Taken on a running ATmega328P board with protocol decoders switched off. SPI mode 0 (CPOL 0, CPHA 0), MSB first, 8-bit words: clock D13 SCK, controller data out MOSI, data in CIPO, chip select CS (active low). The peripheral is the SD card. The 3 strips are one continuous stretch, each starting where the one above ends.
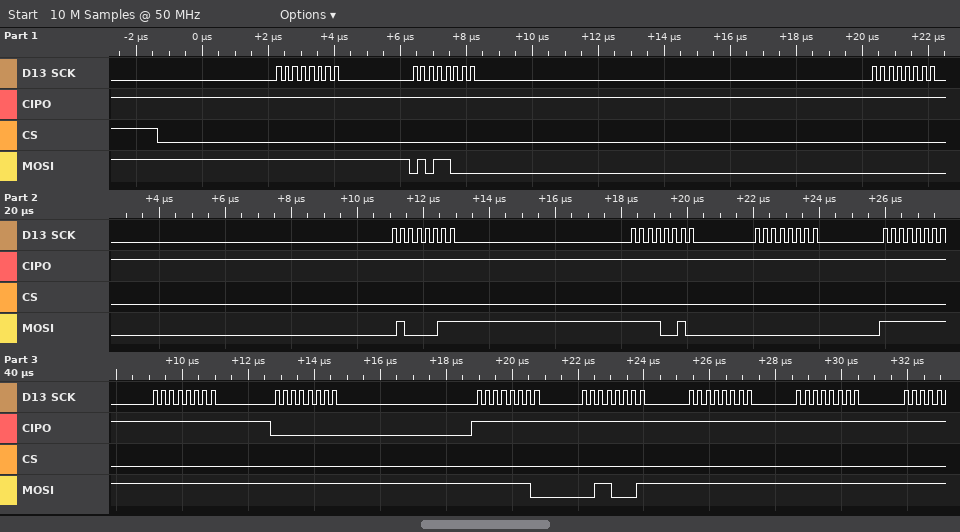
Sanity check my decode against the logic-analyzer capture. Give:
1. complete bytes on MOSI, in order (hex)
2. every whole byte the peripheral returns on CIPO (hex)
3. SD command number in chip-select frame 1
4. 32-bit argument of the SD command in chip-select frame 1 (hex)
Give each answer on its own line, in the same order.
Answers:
FF 58 00 43 F2 00 FF FF FF FE 31 FF FF
FF FF FF FF FF FF FF FF 00 FF FF FF FF
CMD24
0x0043F200
